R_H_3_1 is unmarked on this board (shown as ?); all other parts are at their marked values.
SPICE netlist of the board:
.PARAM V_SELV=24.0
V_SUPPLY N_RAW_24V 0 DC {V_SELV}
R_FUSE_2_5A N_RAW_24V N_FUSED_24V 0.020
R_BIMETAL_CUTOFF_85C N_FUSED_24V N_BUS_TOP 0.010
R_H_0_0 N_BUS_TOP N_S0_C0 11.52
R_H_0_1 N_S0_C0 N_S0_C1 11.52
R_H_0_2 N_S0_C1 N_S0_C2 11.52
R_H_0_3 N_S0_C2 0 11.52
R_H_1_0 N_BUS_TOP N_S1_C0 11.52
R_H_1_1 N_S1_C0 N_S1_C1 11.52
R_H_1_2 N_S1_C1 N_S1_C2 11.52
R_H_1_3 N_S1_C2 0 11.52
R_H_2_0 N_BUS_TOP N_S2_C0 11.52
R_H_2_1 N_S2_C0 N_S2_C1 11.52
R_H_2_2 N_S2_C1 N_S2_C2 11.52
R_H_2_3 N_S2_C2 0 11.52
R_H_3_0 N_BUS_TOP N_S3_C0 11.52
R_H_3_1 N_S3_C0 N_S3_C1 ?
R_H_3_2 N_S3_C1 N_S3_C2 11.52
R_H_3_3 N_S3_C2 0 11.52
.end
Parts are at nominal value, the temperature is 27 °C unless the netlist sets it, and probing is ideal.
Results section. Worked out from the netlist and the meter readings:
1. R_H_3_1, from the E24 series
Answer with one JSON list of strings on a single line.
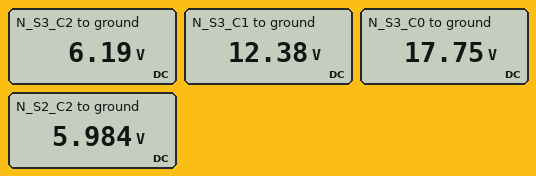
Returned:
["10 Ω"]
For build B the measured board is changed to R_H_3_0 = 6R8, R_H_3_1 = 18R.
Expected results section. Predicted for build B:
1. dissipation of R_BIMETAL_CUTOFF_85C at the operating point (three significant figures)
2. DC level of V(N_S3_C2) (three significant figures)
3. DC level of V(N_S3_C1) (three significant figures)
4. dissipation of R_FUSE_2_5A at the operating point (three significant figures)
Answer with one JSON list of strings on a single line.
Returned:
["42.4 mW", "5.76 V", "11.5 V", "84.8 mW"]
